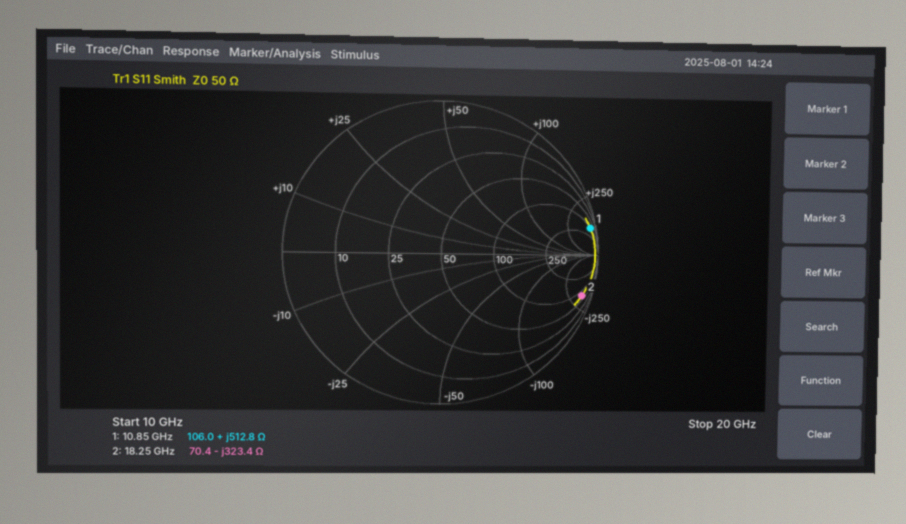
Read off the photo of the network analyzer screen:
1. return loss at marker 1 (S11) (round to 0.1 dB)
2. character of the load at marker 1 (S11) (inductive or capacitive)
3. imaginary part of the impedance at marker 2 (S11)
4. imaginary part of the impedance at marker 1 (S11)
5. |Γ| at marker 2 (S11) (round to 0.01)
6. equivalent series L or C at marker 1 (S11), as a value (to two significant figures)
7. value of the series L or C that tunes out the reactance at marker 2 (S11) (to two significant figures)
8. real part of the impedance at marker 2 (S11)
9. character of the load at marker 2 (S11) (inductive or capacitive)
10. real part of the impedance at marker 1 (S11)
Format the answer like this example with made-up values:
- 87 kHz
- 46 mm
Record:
- 0.3 dB
- inductive
- -323.4 Ω
- +512.8 Ω
- 0.94
- 7.5 nH
- 2.8 nH
- 70.4 Ω
- capacitive
- 106.0 Ω
